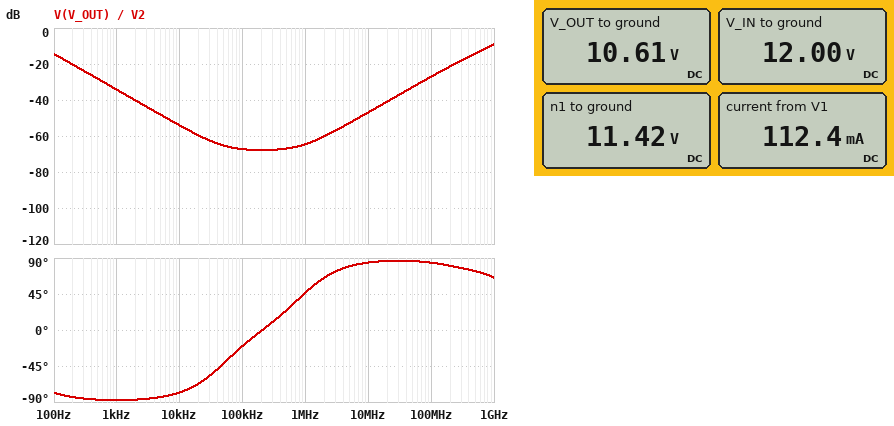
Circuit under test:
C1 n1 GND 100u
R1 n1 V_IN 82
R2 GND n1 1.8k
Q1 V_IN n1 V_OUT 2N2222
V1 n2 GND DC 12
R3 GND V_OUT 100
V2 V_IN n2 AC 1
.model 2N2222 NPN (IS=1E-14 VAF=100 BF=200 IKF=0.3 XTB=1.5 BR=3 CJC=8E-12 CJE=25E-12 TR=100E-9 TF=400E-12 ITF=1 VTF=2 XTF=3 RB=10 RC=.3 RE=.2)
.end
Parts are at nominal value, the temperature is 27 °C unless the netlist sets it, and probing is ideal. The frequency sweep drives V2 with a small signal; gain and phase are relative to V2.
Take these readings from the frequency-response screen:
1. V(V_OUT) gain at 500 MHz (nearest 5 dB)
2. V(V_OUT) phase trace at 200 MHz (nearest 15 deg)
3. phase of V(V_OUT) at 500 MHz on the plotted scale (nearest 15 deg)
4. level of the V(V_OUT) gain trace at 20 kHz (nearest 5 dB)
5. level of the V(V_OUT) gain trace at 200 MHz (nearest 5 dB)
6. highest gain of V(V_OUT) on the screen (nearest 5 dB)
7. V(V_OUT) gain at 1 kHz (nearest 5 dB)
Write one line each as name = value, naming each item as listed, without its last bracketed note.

V(V_OUT) gain at 500 MHz = -15 dB
V(V_OUT) phase trace at 200 MHz = 75 deg
phase of V(V_OUT) at 500 MHz on the plotted scale = 75 deg
level of the V(V_OUT) gain trace at 20 kHz = -60 dB
level of the V(V_OUT) gain trace at 200 MHz = -20 dB
highest gain of V(V_OUT) on the screen = -10 dB
V(V_OUT) gain at 1 kHz = -35 dB
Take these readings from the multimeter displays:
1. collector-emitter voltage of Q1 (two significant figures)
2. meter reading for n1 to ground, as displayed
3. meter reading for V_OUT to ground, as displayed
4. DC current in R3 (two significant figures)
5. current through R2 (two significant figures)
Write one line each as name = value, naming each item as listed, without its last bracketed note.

collector-emitter voltage of Q1 = 1.4 V
meter reading for n1 to ground, as displayed = 11.42 V
meter reading for V_OUT to ground, as displayed = 10.61 V
DC current in R3 = 110 mA
current through R2 = 6.3 mA
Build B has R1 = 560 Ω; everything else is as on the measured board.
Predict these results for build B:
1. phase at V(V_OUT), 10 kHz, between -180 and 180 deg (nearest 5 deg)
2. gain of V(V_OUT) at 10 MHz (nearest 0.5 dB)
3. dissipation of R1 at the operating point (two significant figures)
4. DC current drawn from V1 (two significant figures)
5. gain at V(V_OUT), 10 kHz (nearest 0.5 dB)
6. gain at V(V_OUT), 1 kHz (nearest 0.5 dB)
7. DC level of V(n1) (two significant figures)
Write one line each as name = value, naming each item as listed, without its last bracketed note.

phase at V(V_OUT), 10 kHz, between -180 and 180 deg = -40 deg
gain of V(V_OUT) at 10 MHz = -50.5 dB
dissipation of R1 at the operating point = 17 mW
DC current drawn from V1 = 86 mA
gain at V(V_OUT), 10 kHz = -67.0 dB
gain at V(V_OUT), 1 kHz = -51.0 dB
DC level of V(n1) = 8.9 V
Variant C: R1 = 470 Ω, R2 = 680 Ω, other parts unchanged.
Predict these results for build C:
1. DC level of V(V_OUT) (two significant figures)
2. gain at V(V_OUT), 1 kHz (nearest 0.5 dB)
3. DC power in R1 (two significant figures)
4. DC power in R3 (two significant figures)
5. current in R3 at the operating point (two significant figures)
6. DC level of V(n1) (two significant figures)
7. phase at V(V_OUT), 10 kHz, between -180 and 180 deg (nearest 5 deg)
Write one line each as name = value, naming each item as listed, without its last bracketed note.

DC level of V(V_OUT) = 6.2 V
gain at V(V_OUT), 1 kHz = -49.5 dB
DC power in R1 = 53 mW
DC power in R3 = 390 mW
current in R3 at the operating point = 62 mA
DC level of V(n1) = 7.0 V
phase at V(V_OUT), 10 kHz, between -180 and 180 deg = -45 deg
